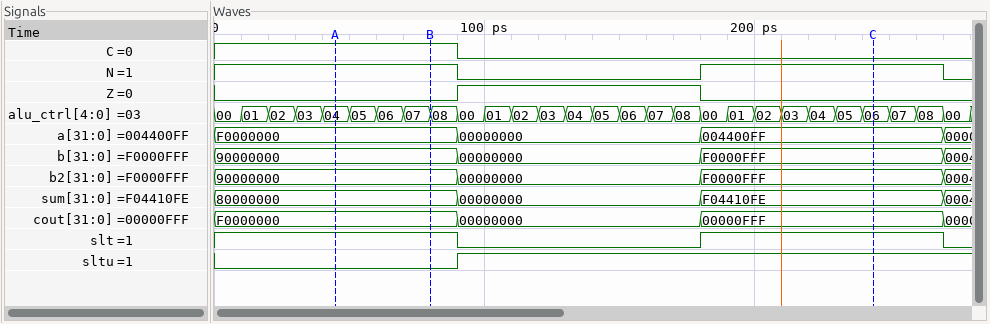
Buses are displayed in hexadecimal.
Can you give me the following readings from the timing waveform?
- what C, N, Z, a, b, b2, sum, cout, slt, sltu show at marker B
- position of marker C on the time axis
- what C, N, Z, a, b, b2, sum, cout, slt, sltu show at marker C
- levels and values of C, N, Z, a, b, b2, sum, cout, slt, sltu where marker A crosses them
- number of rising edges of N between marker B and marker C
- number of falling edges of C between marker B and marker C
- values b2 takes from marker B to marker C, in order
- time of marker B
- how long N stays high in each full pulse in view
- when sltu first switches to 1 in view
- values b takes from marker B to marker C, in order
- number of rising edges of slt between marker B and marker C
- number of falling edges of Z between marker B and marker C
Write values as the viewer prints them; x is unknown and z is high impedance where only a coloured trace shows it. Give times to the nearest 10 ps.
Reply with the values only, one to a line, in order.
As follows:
C=1, N=1, Z=0, a=F0000000, b=90000000, b2=90000000, sum=80000000, cout=F0000000, slt=1, sltu=0
240 ps
C=0, N=1, Z=0, a=004400FF, b=F0000FFF, b2=F0000FFF, sum=F04410FE, cout=00000FFF, slt=1, sltu=1
C=1, N=1, Z=0, a=F0000000, b=90000000, b2=90000000, sum=80000000, cout=F0000000, slt=1, sltu=0
1
1
90000000, 00000000, F0000FFF
80 ps
90 ps
90 ps
90000000, 00000000, F0000FFF
1
1
